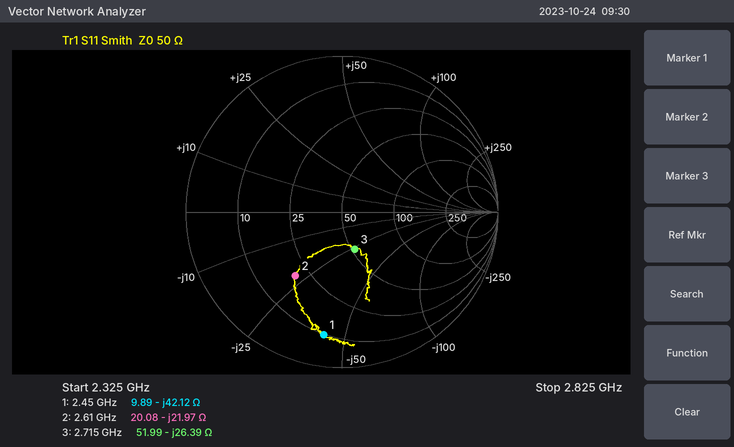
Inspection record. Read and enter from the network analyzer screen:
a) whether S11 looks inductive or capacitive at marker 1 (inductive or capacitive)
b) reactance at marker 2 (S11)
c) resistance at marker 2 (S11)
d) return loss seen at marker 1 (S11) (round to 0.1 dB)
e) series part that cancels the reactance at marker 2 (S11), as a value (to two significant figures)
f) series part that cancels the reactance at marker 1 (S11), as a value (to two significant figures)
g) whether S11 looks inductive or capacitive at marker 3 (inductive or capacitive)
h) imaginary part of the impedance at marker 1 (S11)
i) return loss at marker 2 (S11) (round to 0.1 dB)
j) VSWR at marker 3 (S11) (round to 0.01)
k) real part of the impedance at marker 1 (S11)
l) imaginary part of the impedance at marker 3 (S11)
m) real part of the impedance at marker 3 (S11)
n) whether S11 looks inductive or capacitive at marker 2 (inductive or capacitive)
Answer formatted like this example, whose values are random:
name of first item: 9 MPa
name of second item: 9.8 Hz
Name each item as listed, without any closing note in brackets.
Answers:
whether S11 looks inductive or capacitive at marker 1: capacitive
reactance at marker 2: -21.97 Ω
resistance at marker 2: 20.08 Ω
return loss seen at marker 1 (S11): 2.0 dB
series part that cancels the reactance at marker 2 (S11), as a value: 1.3 nH
series part that cancels the reactance at marker 1 (S11), as a value: 2.7 nH
whether S11 looks inductive or capacitive at marker 3: capacitive
imaginary part of the impedance at marker 1: -42.12 Ω
return loss at marker 2 (S11): 5.9 dB
VSWR at marker 3 (S11): 1.67
real part of the impedance at marker 1: 9.89 Ω
imaginary part of the impedance at marker 3: -26.39 Ω
real part of the impedance at marker 3: 51.99 Ω
whether S11 looks inductive or capacitive at marker 2: capacitive
